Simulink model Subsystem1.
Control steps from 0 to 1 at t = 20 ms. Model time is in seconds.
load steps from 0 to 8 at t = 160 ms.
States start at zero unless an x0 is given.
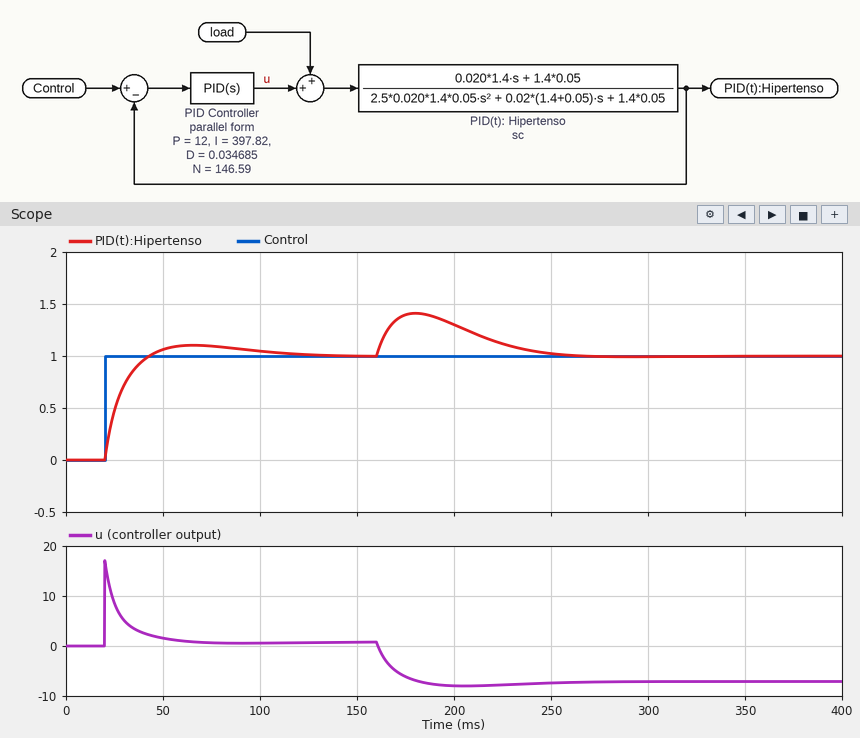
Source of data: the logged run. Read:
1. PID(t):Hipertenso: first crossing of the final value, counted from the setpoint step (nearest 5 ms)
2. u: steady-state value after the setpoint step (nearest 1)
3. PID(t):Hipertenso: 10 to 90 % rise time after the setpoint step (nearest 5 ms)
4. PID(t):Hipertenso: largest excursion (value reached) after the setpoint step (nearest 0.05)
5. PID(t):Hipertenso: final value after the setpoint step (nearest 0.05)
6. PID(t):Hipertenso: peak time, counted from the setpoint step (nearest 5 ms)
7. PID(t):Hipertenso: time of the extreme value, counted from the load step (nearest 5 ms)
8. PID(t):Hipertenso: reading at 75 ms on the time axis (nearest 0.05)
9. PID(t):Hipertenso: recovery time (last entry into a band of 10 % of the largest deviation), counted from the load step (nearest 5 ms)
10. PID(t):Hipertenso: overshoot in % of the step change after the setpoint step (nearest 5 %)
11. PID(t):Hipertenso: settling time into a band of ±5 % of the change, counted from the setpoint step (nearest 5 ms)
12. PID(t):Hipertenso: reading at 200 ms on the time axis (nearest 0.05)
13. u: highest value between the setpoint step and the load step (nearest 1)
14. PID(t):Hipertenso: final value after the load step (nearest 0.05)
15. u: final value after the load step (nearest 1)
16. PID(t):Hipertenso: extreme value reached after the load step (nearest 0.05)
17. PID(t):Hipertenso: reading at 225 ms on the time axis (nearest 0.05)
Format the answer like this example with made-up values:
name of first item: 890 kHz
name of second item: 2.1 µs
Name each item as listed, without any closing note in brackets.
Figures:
PID(t):Hipertenso: first crossing of the final value, counted from the setpoint step: 25 ms
u: steady-state value after the setpoint step: 1
PID(t):Hipertenso: 10 to 90 % rise time after the setpoint step: 15 ms
PID(t):Hipertenso: largest excursion (value reached) after the setpoint step: 1.10
PID(t):Hipertenso: final value after the setpoint step: 1.00
PID(t):Hipertenso: peak time, counted from the setpoint step: 45 ms
PID(t):Hipertenso: time of the extreme value, counted from the load step: 20 ms
PID(t):Hipertenso: reading at 75 ms on the time axis: 1.10
PID(t):Hipertenso: recovery time (last entry into a band of 10 % of the largest deviation), counted from the load step: 85 ms
PID(t):Hipertenso: overshoot in % of the step change after the setpoint step: 10 %
PID(t):Hipertenso: settling time into a band of ±5 % of the change, counted from the setpoint step: 80 ms
PID(t):Hipertenso: reading at 200 ms on the time axis: 1.30
u: highest value between the setpoint step and the load step: 17
PID(t):Hipertenso: final value after the load step: 1.00
u: final value after the load step: -7
PID(t):Hipertenso: extreme value reached after the load step: 1.40
PID(t):Hipertenso: reading at 225 ms on the time axis: 1.10
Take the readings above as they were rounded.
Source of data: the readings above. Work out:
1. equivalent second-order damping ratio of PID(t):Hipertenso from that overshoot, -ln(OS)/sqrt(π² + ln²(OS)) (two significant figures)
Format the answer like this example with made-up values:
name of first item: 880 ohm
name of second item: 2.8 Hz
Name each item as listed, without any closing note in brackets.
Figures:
equivalent second-order damping ratio of PID(t):Hipertenso from that overshoot, -ln(OS)/sqrt(π² + ln²(OS)): 0.59
